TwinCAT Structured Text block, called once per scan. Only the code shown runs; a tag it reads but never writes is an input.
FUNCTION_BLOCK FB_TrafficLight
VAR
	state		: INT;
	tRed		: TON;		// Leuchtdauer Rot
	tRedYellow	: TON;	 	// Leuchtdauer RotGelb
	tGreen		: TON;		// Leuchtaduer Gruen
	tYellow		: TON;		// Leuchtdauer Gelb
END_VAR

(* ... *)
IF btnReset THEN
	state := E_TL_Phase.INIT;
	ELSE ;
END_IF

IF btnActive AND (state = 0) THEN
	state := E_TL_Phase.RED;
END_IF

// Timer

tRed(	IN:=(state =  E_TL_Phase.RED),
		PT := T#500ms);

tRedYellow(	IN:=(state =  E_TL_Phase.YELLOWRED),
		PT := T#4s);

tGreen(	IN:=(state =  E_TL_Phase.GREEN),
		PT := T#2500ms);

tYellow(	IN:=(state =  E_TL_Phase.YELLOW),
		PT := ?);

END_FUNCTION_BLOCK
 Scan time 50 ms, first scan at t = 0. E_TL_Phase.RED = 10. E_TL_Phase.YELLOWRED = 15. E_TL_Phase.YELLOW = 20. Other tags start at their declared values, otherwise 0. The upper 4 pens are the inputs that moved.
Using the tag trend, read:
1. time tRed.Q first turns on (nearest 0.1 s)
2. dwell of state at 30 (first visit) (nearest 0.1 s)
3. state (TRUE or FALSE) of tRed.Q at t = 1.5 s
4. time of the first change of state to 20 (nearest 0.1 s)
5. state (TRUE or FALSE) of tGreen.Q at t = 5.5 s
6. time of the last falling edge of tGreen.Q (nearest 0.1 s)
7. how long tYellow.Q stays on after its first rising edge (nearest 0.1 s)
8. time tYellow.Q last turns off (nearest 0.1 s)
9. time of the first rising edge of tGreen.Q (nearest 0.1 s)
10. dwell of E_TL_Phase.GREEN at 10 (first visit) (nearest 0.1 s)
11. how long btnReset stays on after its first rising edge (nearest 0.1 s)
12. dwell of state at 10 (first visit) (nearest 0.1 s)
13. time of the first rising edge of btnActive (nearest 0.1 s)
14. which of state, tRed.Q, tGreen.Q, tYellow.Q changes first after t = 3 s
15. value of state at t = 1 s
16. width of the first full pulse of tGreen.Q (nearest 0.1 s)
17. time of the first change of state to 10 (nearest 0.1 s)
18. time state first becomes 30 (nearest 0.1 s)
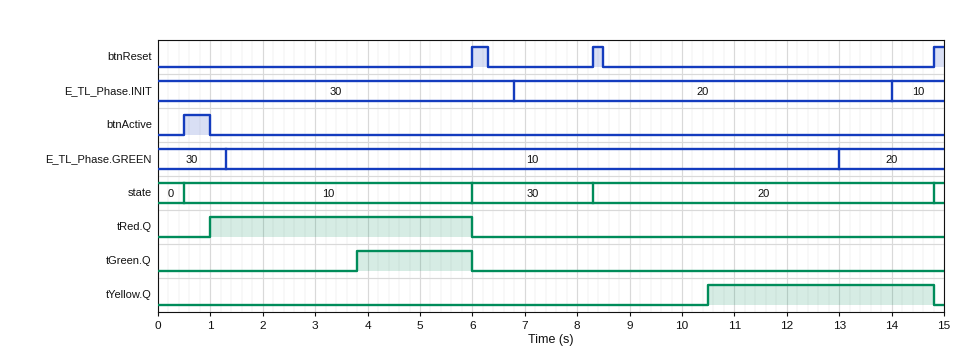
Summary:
1.0 s
2.3 s
TRUE
8.3 s
TRUE
6.0 s
4.3 s
14.8 s
3.8 s
11.7 s
0.3 s
5.5 s
0.5 s
tGreen.Q
10
2.2 s
0.5 s
6.0 s
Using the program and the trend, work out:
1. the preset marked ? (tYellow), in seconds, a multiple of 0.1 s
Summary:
2.2 s
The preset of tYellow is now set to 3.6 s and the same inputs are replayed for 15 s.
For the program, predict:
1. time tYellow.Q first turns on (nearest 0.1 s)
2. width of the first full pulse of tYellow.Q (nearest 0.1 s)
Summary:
11.9 s
2.9 s
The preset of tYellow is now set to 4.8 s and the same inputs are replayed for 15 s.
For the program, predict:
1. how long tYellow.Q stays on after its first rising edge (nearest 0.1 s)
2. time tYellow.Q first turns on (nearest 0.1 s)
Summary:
1.7 s
13.1 s
